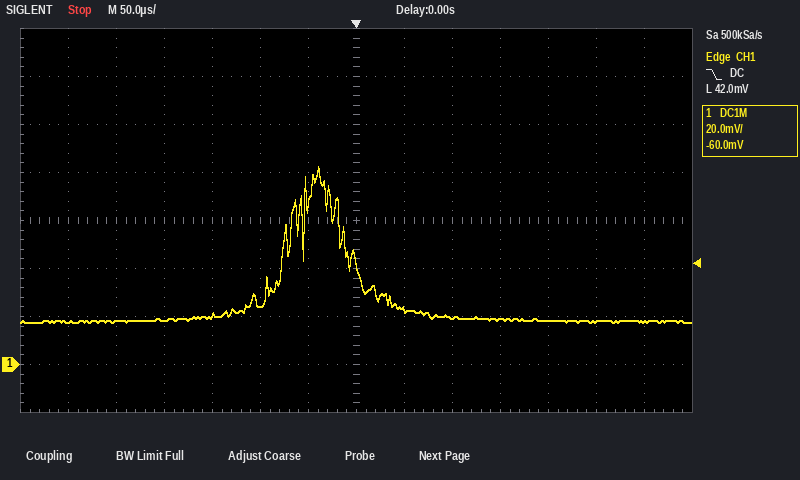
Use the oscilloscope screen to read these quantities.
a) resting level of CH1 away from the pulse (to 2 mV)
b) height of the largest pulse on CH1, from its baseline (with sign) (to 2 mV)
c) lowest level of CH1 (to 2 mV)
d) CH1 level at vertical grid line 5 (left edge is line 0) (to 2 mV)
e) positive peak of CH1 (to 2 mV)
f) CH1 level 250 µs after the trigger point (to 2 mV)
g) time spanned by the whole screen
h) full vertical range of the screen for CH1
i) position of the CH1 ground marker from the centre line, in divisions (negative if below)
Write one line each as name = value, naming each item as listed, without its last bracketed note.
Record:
resting level of CH1 away from the pulse = 18 mV
height of the largest pulse on CH1, from its baseline (with sign) = +64 mV
lowest level of CH1 = 18 mV
CH1 level at vertical grid line 5 (left edge is line 0) = 24 mV
positive peak of CH1 = 82 mV
CH1 level 250 µs after the trigger point = 18 mV
time spanned by the whole screen = 700 µs
full vertical range of the screen for CH1 = 160 mV
position of the CH1 ground marker from the centre line, in divisions = -3.0 div
